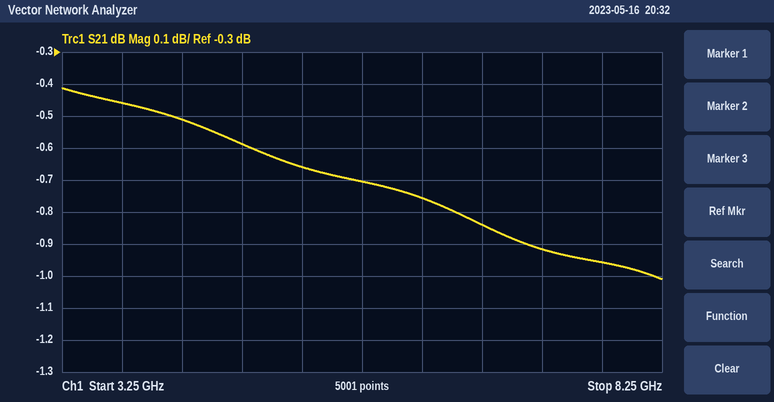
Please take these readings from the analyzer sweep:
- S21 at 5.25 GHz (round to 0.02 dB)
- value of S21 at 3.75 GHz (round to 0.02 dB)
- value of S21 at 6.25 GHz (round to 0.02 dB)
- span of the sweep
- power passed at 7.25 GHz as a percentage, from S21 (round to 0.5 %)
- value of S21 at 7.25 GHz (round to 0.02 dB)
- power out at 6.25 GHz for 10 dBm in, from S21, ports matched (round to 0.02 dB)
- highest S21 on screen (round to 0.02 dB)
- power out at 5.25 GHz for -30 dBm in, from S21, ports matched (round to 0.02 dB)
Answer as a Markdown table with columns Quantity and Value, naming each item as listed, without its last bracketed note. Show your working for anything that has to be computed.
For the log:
| Quantity | Value |
|---|---|
| S21 at 5.25 GHz | -0.66 dB |
| value of S21 at 3.75 GHz | -0.46 dB |
| value of S21 at 6.25 GHz | -0.76 dB |
| span of the sweep | 5 GHz |
| power passed at 7.25 GHz as a percentage, from S21 | 10^(-0.92/10) ≈ 80.9 %, so 81.0 % to the nearest 0.5 % |
| value of S21 at 7.25 GHz | -0.92 dB |
| power out at 6.25 GHz for 10 dBm in, from S21, ports matched | 10 dBm + (-0.76 dB) = 9.24 dBm |
| highest S21 on screen | -0.42 dB |
| power out at 5.25 GHz for -30 dBm in, from S21, ports matched | -30 dBm + (-0.66 dB) = -30.66 dBm |
